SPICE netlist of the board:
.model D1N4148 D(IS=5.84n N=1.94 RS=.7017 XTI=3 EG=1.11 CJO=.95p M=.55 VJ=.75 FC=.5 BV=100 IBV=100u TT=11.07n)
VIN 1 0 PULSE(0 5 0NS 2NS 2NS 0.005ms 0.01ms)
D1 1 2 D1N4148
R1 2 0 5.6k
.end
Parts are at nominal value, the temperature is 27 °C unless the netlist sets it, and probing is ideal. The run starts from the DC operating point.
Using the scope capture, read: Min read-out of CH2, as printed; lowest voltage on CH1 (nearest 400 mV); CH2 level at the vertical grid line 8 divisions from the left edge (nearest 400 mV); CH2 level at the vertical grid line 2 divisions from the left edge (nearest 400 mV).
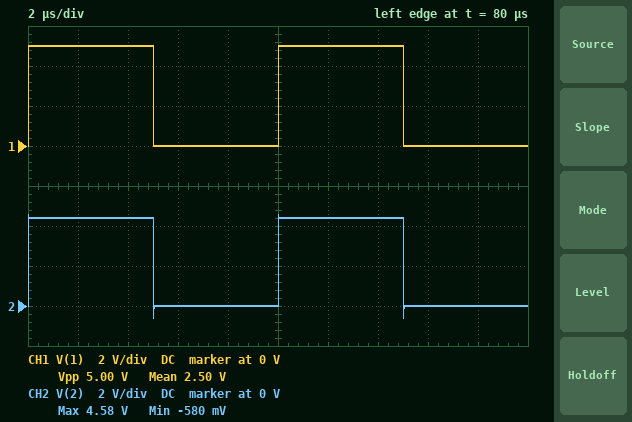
-580 mV
0 V
0 V
4.4 V
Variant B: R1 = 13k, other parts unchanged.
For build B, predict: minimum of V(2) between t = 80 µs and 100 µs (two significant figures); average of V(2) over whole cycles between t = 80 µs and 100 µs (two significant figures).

-550 mV
2.2 V
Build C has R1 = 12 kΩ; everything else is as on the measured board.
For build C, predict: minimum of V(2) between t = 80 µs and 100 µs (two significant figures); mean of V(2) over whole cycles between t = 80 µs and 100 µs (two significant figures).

-550 mV
2.2 V
